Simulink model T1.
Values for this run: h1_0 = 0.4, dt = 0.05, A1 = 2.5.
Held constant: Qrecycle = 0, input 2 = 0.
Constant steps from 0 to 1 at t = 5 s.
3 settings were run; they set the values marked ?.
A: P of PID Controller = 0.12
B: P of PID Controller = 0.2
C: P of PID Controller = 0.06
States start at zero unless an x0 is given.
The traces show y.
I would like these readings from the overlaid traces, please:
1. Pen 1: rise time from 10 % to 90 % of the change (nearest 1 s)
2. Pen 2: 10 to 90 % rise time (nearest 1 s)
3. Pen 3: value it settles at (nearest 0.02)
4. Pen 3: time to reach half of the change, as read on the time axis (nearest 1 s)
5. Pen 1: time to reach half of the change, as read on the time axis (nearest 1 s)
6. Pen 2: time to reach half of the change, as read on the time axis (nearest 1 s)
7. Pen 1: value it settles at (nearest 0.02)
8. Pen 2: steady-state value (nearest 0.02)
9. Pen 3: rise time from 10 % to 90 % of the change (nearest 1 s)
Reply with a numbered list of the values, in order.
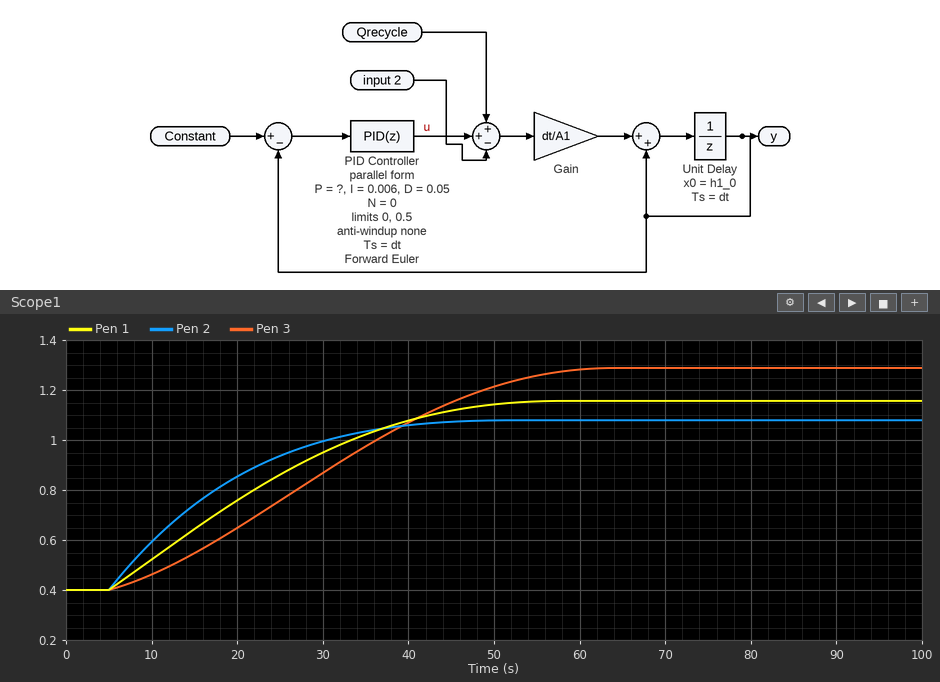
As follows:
1. 32 s
2. 25 s
3. 1.28
4. 29 s
5. 21 s
6. 15 s
7. 1.16
8. 1.08
9. 37 s
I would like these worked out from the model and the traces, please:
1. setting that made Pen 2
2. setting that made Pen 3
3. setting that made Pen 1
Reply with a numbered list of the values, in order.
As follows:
1. B
2. C
3. A
